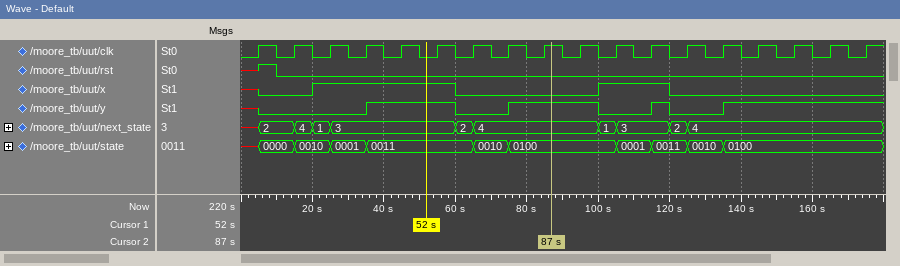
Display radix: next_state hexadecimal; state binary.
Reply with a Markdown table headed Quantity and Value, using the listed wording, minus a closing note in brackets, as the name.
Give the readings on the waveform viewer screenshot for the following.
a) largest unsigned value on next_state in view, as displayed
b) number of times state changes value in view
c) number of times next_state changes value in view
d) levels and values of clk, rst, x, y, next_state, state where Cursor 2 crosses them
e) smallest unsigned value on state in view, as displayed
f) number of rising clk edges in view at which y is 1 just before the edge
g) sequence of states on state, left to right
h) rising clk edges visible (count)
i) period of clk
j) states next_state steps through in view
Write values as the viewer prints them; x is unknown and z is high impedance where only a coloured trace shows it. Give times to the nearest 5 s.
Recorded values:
| Quantity | Value |
|---|---|
| largest unsigned value on next_state in view, as displayed | 4 |
| number of times state changes value in view | 10 |
| number of times next_state changes value in view | 10 |
| levels and values of clk, rst, x, y, next_state, state where Cursor 2 crosses them | clk=1, rst=0, x=0, y=1, next_state=4, state=0100 |
| smallest unsigned value on state in view, as displayed | 0000 |
| number of rising clk edges in view at which y is 1 just before the edge | 8 |
| sequence of states on state, left to right | x, 0000, 0010, 0001, 0011, 0010, 0100, 0001, 0011, 0010, 0100 |
| rising clk edges visible | 18 |
| period of clk | 10 s |
| states next_state steps through in view | x, 2, 4, 1, 3, 2, 4, 1, 3, 2, 4 |
